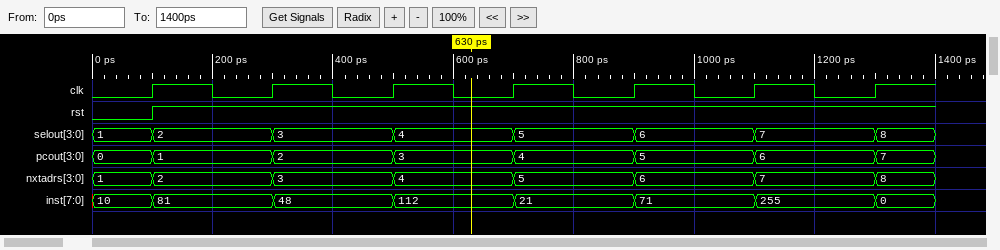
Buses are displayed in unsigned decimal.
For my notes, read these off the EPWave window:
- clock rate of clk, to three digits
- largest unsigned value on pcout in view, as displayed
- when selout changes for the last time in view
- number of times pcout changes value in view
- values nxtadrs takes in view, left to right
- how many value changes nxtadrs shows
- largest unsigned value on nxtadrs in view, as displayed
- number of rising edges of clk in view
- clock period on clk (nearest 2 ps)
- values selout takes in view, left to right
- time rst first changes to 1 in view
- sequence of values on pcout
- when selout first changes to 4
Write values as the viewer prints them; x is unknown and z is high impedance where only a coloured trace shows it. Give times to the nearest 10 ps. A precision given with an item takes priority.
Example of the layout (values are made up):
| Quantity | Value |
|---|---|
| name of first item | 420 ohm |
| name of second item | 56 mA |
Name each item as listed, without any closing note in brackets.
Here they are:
| Quantity | Value |
|---|---|
| clock rate of clk, to three digits | 5.00 GHz |
| largest unsigned value on pcout in view, as displayed | 7 |
| when selout changes for the last time in view | 1300 ps |
| number of times pcout changes value in view | 7 |
| values nxtadrs takes in view, left to right | 1, 2, 3, 4, 5, 6, 7, 8 |
| how many value changes nxtadrs shows | 7 |
| largest unsigned value on nxtadrs in view, as displayed | 8 |
| number of rising edges of clk in view | 7 |
| clock period on clk | 200 ps |
| values selout takes in view, left to right | 1, 2, 3, 4, 5, 6, 7, 8 |
| time rst first changes to 1 in view | 100 ps |
| sequence of values on pcout | 0, 1, 2, 3, 4, 5, 6, 7 |
| when selout first changes to 4 | 500 ps |
